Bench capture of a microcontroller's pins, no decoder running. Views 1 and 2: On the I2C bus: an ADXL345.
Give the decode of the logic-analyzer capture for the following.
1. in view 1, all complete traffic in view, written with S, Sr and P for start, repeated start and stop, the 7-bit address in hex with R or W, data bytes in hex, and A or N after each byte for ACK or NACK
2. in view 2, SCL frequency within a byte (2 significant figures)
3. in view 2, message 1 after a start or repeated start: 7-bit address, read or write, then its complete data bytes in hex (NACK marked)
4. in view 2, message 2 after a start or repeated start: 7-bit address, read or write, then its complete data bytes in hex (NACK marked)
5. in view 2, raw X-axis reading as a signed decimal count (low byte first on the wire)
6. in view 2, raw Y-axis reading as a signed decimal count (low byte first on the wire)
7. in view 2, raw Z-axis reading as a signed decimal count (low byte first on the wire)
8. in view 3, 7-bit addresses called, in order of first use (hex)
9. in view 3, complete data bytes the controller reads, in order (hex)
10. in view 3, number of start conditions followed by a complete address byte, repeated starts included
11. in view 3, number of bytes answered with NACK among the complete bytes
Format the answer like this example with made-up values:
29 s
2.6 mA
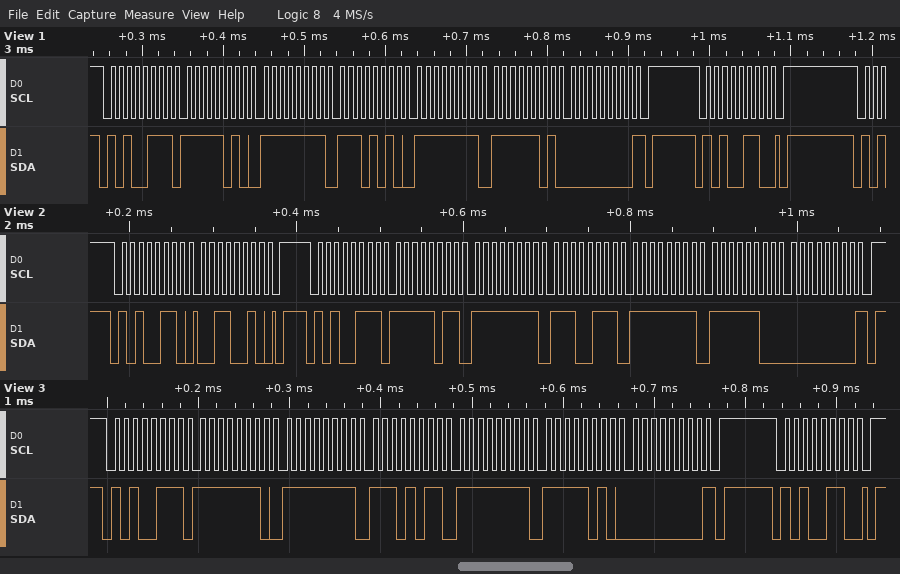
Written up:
S 53R A FA A FF A EA A FF A FD A 00 N P S 53W A P
100 kHz
0x53 write: 32
0x53 read: FB FF E7 FF FC 00 NACK
-5
-25
252
0x53
FE FF EB FF FA 00
2
1
